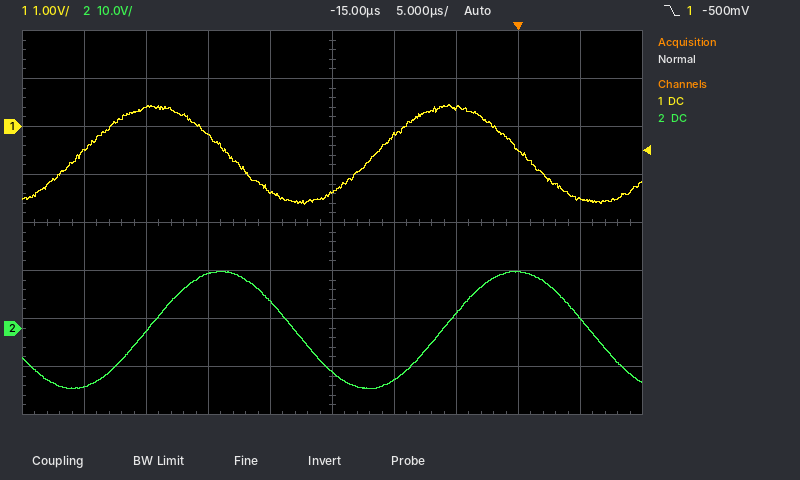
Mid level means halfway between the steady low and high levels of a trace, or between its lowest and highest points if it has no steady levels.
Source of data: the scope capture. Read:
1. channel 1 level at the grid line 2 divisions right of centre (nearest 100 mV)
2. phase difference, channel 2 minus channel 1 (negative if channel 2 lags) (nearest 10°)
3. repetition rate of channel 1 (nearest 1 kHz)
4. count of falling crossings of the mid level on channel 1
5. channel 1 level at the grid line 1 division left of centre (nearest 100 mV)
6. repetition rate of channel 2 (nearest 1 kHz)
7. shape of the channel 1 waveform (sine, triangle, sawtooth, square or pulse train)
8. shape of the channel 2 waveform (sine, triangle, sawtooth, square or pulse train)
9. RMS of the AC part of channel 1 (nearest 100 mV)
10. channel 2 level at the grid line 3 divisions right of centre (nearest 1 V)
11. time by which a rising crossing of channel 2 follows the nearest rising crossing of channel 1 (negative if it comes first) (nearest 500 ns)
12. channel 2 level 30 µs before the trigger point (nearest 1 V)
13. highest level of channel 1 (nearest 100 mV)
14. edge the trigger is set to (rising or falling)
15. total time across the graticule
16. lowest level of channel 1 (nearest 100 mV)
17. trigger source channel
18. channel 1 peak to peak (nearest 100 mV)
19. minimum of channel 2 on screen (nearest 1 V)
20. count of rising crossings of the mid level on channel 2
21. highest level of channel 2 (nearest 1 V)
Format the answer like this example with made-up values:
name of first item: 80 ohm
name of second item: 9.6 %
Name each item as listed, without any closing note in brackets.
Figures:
channel 1 level at the grid line 2 divisions right of centre: 400 mV
phase difference, channel 2 minus channel 1 (negative if channel 2 lags): -80°
repetition rate of channel 1: 42 kHz
count of falling crossings of the mid level on channel 1: 2
channel 1 level at the grid line 1 division left of centre: -1.4 V
repetition rate of channel 2: 42 kHz
shape of the channel 1 waveform: sine
shape of the channel 2 waveform: sine
RMS of the AC part of channel 1: 700 mV
channel 2 level at the grid line 3 divisions right of centre: 12 V
time by which a rising crossing of channel 2 follows the nearest rising crossing of channel 1 (negative if it comes first): +5.5 µs
channel 2 level 30 µs before the trigger point: -1 V
highest level of channel 1: 500 mV
edge the trigger is set to: falling
total time across the graticule: 50 µs
lowest level of channel 1: -1.6 V
trigger source channel: channel 1
channel 1 peak to peak: 2.1 V
minimum of channel 2 on screen: -13 V
count of rising crossings of the mid level on channel 2: 2
highest level of channel 2: 12 V
